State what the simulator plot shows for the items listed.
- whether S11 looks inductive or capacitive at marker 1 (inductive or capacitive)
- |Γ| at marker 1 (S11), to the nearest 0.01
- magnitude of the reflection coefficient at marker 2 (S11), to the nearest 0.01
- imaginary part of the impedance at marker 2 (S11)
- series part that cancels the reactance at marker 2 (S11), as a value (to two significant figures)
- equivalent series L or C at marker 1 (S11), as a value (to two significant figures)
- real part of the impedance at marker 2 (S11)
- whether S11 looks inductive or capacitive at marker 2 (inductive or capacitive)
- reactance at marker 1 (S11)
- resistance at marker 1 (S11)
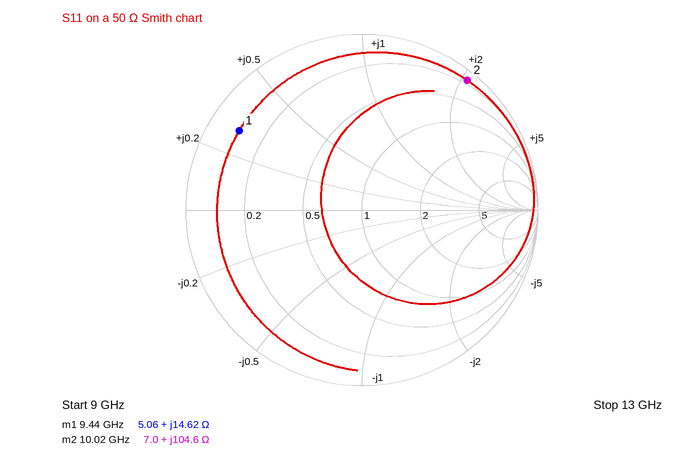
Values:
inductive
0.83
0.95
+104.6 Ω
150 fF
250 pH
7.0 Ω
inductive
+14.62 Ω
5.06 Ω
